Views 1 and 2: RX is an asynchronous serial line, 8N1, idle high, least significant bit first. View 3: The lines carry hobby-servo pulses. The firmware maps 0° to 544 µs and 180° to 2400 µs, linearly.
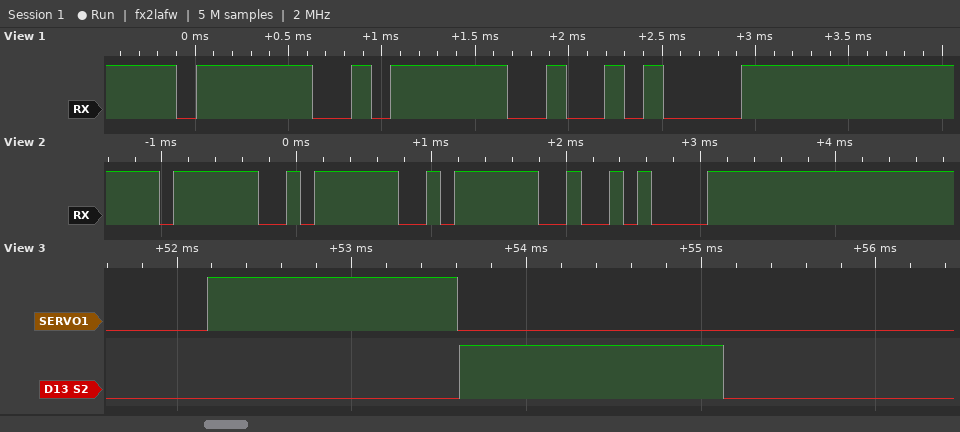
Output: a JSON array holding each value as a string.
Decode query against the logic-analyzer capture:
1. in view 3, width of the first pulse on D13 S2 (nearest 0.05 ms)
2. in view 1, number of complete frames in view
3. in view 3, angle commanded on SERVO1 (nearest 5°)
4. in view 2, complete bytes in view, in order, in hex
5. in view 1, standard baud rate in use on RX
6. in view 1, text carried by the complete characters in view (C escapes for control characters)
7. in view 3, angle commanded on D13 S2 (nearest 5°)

["1.50 ms", "3", "85°", "3F 3F 3F 0A", "9600 baud", "\"??\\n\"", "95°"]
